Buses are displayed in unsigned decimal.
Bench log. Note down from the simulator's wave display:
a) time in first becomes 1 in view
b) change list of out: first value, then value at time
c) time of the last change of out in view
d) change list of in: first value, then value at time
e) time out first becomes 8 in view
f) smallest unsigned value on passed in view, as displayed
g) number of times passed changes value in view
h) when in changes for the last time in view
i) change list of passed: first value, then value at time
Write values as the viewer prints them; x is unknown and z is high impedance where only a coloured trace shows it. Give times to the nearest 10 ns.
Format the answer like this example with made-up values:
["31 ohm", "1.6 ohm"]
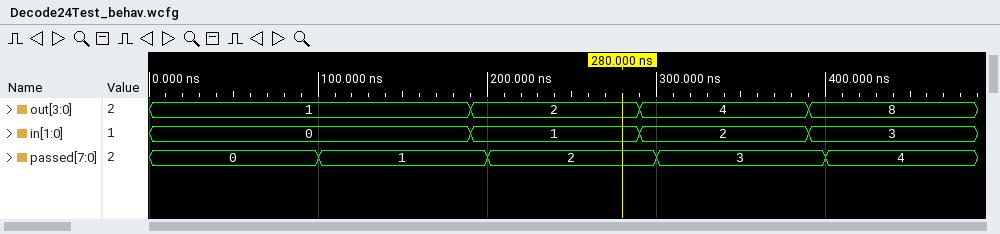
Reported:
["190 ns", "1, 2 at 190 ns, 4 at 290 ns, 8 at 390 ns", "390 ns", "0, 1 at 190 ns, 2 at 290 ns, 3 at 390 ns", "390 ns", "0", "4", "390 ns", "0, 1 at 100 ns, 2 at 200 ns, 3 at 300 ns, 4 at 400 ns"]
